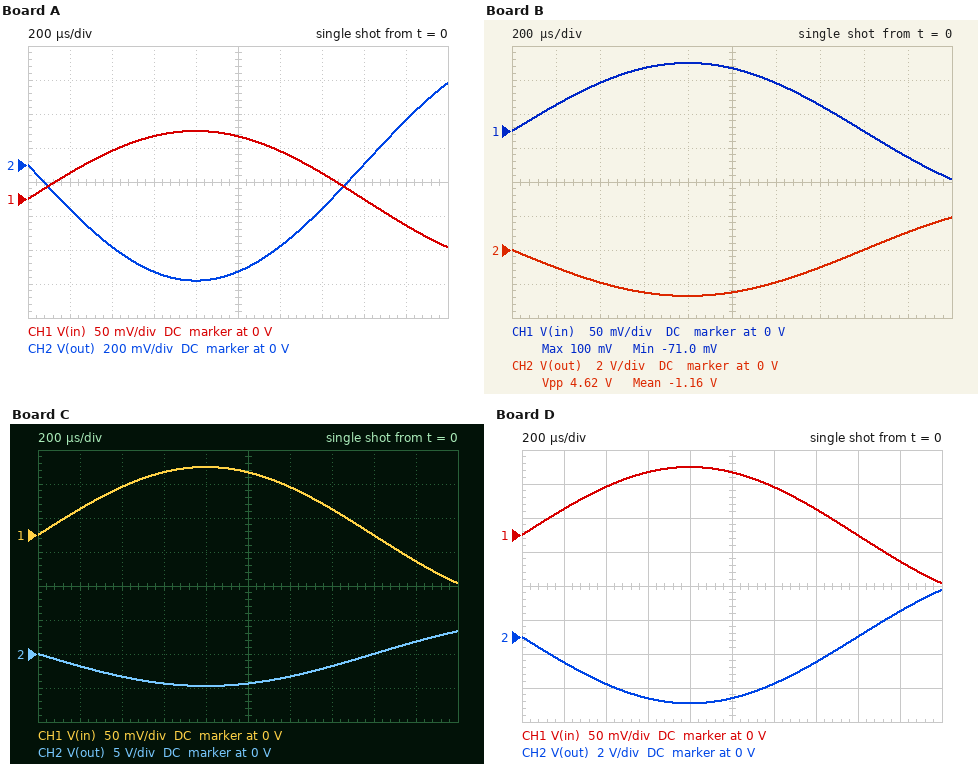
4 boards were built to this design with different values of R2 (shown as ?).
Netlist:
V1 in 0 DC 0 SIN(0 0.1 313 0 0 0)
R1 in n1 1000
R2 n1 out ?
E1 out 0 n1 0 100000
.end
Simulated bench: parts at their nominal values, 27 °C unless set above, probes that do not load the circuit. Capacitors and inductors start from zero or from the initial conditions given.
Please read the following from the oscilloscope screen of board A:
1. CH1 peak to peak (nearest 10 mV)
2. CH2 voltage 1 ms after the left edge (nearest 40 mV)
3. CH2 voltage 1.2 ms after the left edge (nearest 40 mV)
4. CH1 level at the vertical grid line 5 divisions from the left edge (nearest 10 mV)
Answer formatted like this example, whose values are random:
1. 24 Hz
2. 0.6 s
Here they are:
1. 170 mV
2. -640 mV
3. -480 mV
4. 90 mV
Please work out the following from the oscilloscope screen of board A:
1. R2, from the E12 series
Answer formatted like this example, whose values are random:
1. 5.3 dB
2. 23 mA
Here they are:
1. 6.8 kΩ
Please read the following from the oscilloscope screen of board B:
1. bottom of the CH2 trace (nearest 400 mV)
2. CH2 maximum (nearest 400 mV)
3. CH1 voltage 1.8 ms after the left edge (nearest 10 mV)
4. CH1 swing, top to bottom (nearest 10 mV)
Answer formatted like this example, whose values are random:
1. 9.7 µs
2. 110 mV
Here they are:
1. -2.8 V
2. 2.0 V
3. -40 mV
4. 170 mV
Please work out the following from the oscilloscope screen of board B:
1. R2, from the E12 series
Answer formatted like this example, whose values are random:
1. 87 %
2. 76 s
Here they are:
1. 27 kΩ
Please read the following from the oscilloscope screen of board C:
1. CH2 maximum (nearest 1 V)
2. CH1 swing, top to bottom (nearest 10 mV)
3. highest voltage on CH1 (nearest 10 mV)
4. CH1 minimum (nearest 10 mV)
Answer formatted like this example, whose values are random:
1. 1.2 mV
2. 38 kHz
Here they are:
1. 3 V
2. 170 mV
3. 100 mV
4. -70 mV
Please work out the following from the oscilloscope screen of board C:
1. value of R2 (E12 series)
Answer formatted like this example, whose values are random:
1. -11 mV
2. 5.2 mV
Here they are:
1. 47 kΩ
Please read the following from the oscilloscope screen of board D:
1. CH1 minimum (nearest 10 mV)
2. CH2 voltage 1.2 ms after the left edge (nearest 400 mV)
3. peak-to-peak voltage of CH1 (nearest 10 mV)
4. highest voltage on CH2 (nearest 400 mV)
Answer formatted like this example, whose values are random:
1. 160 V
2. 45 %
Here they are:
1. -70 mV
2. -2.8 V
3. 170 mV
4. 2.8 V
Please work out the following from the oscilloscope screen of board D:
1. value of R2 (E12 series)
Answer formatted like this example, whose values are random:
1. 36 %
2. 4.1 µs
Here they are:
1. 39 kΩ
